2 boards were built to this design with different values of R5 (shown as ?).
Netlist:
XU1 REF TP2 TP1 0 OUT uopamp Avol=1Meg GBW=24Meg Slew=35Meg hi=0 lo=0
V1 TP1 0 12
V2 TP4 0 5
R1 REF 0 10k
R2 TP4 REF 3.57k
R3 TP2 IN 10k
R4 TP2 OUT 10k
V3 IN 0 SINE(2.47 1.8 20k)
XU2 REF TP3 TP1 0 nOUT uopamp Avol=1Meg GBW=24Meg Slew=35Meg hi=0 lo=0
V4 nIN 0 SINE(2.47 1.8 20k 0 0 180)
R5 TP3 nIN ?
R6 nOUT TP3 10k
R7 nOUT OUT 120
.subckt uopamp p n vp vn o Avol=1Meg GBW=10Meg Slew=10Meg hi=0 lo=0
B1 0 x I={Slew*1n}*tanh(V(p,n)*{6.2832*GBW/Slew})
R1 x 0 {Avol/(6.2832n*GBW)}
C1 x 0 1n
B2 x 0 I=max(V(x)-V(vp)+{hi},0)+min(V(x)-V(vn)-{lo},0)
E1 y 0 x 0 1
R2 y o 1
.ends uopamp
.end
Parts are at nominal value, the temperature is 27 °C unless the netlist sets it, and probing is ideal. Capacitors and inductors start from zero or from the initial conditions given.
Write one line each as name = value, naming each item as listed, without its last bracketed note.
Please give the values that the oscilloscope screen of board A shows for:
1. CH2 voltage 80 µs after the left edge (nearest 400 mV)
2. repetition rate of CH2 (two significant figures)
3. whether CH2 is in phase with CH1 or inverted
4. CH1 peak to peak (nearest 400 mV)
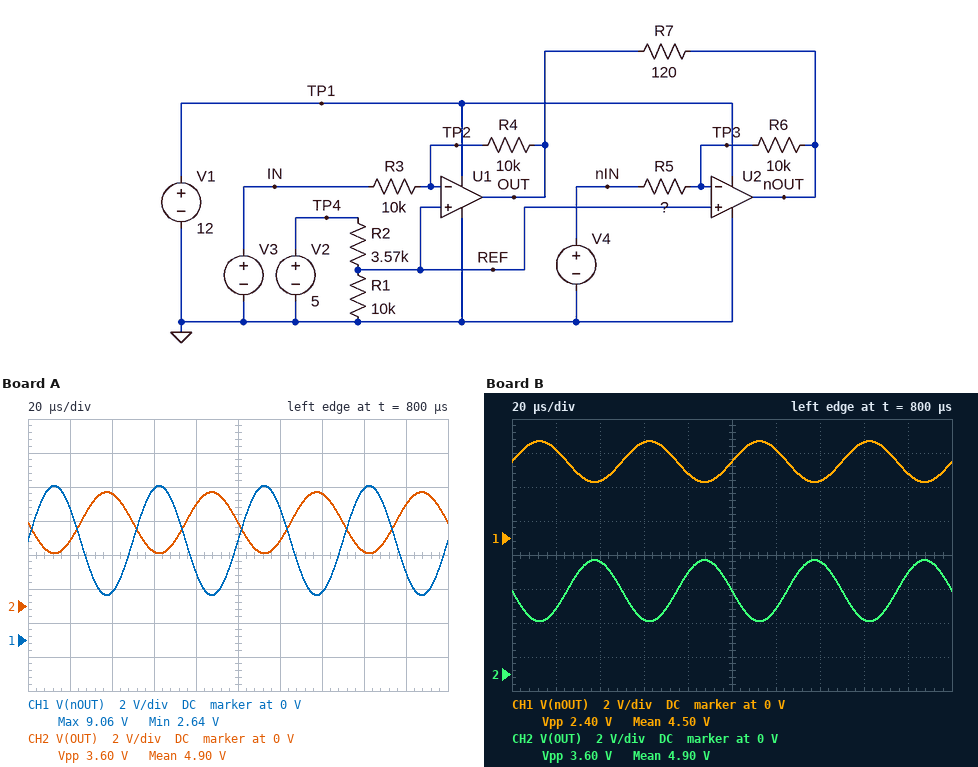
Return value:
CH2 voltage 80 µs after the left edge = 6.0 V
repetition rate of CH2 = 20 kHz
whether CH2 is in phase with CH1 or inverted = inverted
CH1 peak to peak = 6.4 V
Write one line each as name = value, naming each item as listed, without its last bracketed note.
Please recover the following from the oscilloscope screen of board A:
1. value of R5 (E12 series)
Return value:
value of R5 = 5.6 kΩ
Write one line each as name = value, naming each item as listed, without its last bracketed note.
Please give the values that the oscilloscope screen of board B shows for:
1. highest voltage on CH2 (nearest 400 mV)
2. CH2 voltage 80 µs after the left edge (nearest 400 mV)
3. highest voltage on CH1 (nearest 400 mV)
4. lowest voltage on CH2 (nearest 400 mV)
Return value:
highest voltage on CH2 = 6.8 V
CH2 voltage 80 µs after the left edge = 6.0 V
highest voltage on CH1 = 5.6 V
lowest voltage on CH2 = 3.2 V
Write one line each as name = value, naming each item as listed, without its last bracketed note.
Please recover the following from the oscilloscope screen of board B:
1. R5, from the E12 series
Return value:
R5, from the E12 series = 15 kΩ
